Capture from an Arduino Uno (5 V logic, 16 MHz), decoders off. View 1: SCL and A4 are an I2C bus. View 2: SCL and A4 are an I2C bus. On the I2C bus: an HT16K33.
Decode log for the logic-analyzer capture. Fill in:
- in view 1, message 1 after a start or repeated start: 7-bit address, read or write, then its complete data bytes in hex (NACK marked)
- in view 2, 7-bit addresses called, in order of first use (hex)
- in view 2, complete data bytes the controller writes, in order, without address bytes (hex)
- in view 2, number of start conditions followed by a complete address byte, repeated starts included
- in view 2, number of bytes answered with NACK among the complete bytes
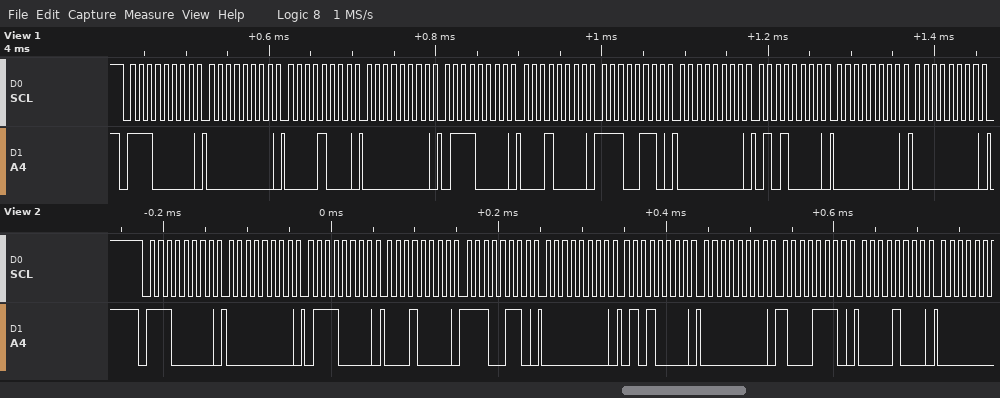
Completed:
0x70 write: 00 08 00 70 10 E6 00 50 00 00
0x70
00 70 10 E6 00 50 00 8E 08
1
0
